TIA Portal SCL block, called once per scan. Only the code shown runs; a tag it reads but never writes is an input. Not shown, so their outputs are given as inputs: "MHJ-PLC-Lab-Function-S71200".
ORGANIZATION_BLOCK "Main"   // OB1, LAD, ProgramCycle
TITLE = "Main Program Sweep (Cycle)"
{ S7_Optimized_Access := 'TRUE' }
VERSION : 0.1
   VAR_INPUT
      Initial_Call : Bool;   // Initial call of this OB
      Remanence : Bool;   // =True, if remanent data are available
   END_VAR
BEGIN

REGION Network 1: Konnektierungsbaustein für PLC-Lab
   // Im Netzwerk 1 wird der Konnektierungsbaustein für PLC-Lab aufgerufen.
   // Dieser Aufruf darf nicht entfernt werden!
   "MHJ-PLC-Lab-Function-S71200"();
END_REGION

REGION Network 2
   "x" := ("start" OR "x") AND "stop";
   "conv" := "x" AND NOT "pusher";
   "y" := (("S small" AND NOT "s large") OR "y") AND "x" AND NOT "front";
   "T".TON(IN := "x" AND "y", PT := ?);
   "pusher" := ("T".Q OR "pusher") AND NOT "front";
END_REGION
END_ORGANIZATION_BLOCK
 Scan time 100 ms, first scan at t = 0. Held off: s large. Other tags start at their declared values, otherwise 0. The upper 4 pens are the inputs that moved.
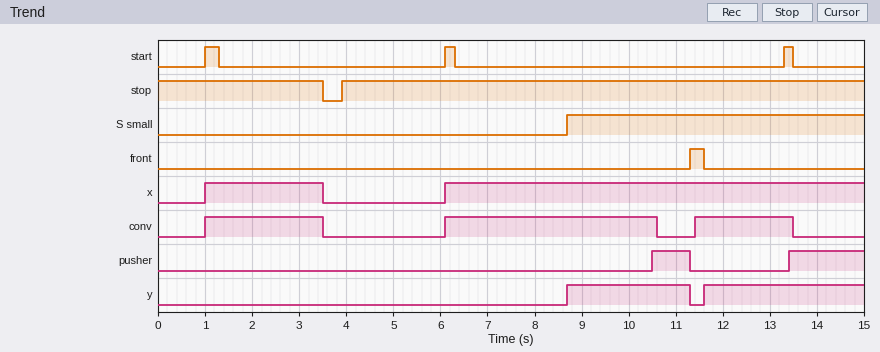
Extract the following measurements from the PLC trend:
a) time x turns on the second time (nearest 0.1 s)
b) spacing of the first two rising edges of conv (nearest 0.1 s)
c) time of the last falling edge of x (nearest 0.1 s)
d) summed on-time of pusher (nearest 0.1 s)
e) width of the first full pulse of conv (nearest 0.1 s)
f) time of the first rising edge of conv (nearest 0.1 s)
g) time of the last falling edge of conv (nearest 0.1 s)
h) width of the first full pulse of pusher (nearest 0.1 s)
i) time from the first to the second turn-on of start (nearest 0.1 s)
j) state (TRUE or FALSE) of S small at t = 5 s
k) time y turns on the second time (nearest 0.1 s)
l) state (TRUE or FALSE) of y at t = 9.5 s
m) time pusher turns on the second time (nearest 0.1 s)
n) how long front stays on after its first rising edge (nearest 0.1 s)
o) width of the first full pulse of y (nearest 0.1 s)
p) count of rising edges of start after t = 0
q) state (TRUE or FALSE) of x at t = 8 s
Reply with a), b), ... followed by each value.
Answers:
a) 6.1 s
b) 5.1 s
c) 3.5 s
d) 2.4 s
e) 2.5 s
f) 1.0 s
g) 13.5 s
h) 0.8 s
i) 5.1 s
j) FALSE
k) 11.6 s
l) TRUE
m) 13.4 s
n) 0.3 s
o) 2.6 s
p) 3
q) TRUE
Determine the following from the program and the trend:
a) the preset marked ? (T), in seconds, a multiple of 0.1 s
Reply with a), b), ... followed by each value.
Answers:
a) 1.8 s
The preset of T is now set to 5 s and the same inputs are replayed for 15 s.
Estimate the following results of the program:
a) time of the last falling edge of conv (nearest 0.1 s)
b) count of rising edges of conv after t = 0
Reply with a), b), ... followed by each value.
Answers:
a) 3.5 s
b) 2
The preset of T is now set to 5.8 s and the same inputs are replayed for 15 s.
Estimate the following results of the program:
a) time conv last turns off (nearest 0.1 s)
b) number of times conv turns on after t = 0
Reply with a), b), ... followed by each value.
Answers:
a) 3.5 s
b) 2
